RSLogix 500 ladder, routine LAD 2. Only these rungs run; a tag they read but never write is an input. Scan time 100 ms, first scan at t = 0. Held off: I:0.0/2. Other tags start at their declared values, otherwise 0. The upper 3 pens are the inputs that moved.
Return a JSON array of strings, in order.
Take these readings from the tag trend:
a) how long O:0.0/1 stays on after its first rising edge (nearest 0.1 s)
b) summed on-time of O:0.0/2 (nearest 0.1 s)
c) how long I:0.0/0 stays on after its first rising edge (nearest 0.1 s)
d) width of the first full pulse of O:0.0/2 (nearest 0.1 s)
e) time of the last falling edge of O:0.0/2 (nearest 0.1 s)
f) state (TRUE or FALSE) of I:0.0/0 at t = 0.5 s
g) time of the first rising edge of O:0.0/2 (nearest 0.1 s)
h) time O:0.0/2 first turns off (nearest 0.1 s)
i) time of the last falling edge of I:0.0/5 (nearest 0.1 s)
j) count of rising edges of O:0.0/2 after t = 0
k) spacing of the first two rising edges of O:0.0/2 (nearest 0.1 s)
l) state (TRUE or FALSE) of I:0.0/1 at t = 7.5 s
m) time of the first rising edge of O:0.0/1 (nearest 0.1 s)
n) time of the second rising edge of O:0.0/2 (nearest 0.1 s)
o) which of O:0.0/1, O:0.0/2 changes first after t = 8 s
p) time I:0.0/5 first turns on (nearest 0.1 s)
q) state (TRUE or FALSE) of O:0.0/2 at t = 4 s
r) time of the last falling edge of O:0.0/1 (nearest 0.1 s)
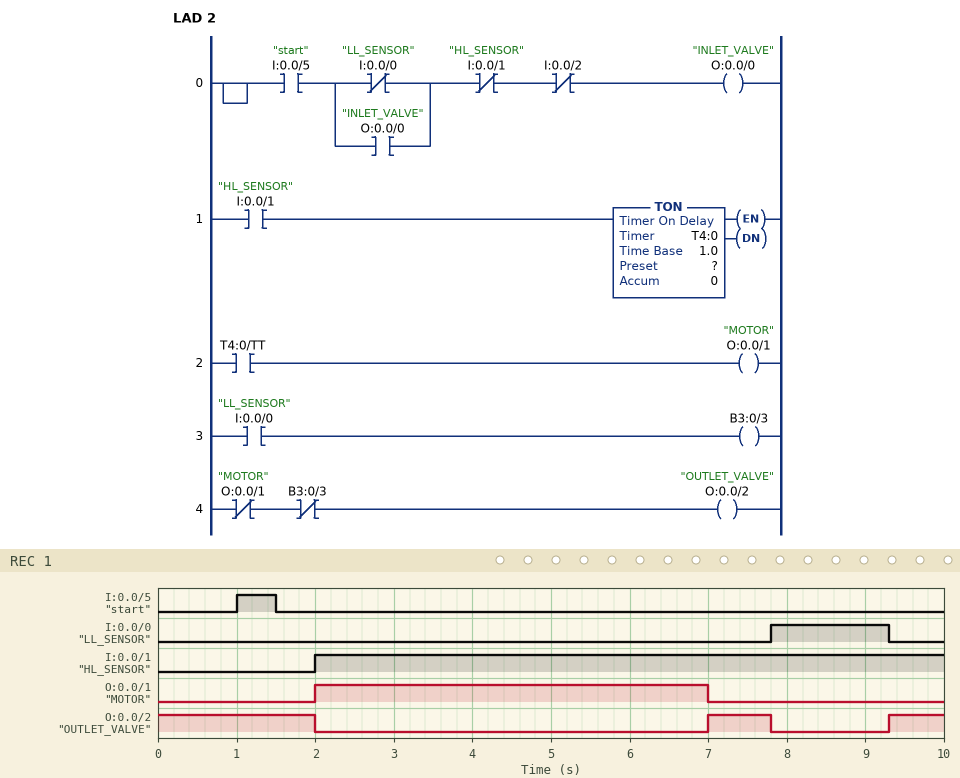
["5.0 s", "3.5 s", "1.5 s", "0.8 s", "7.8 s", "FALSE", "7.0 s", "2.0 s", "1.5 s", "2", "2.3 s", "TRUE", "2.0 s", "9.3 s", "O:0.0/2", "1.0 s", "FALSE", "7.0 s"]
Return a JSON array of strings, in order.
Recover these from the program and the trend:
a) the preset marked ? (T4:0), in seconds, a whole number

["5 s"]
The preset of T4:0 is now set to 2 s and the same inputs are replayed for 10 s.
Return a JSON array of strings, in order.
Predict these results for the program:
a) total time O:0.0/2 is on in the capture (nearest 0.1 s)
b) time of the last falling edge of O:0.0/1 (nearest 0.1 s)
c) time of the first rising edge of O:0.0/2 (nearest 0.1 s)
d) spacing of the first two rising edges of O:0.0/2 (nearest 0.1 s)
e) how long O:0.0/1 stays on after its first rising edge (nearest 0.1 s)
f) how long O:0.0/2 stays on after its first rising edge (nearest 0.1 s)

["6.5 s", "4.0 s", "4.0 s", "5.3 s", "2.0 s", "3.8 s"]
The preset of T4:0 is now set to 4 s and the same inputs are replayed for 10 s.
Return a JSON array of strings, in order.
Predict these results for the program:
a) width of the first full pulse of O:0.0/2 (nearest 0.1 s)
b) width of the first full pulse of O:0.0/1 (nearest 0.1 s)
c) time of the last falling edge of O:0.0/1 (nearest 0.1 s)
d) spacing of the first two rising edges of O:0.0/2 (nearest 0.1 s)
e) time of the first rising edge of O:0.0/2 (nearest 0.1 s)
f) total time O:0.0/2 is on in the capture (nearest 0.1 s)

["1.8 s", "4.0 s", "6.0 s", "3.3 s", "6.0 s", "4.5 s"]
